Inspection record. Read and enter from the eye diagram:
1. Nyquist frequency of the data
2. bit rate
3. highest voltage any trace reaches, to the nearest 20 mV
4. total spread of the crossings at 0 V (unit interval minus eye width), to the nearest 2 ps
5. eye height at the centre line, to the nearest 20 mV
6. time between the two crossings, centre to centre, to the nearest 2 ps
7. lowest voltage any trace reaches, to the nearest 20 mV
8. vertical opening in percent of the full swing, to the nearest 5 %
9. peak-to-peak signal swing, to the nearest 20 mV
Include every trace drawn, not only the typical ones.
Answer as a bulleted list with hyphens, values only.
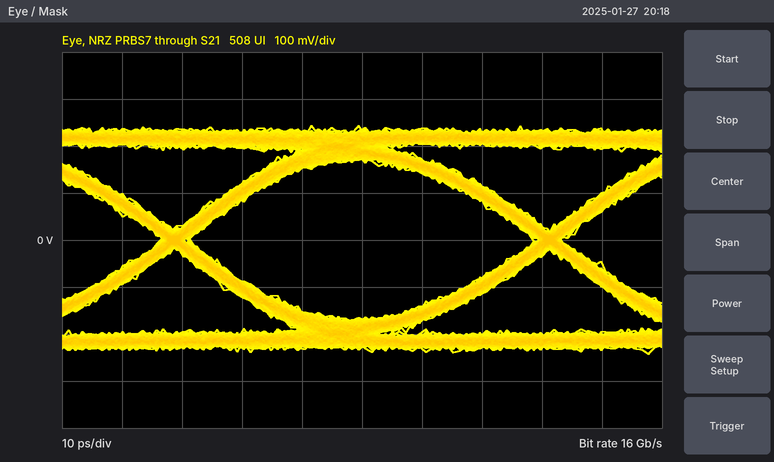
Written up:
- 8 GHz
- 16 Gb/s
- 240 mV
- 6 ps
- 340 mV
- 62 ps
- -240 mV
- 70 %
- 480 mV
